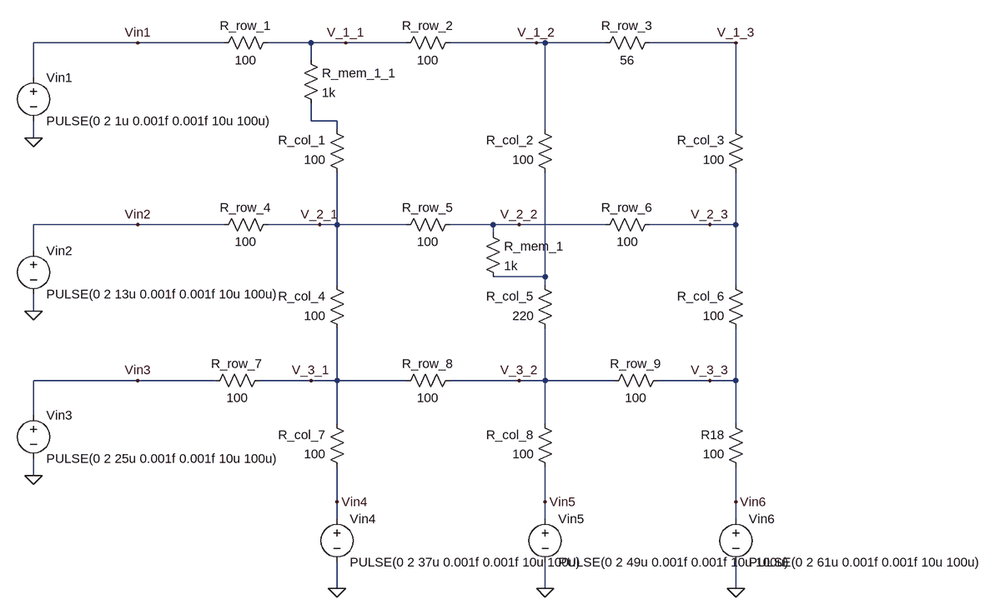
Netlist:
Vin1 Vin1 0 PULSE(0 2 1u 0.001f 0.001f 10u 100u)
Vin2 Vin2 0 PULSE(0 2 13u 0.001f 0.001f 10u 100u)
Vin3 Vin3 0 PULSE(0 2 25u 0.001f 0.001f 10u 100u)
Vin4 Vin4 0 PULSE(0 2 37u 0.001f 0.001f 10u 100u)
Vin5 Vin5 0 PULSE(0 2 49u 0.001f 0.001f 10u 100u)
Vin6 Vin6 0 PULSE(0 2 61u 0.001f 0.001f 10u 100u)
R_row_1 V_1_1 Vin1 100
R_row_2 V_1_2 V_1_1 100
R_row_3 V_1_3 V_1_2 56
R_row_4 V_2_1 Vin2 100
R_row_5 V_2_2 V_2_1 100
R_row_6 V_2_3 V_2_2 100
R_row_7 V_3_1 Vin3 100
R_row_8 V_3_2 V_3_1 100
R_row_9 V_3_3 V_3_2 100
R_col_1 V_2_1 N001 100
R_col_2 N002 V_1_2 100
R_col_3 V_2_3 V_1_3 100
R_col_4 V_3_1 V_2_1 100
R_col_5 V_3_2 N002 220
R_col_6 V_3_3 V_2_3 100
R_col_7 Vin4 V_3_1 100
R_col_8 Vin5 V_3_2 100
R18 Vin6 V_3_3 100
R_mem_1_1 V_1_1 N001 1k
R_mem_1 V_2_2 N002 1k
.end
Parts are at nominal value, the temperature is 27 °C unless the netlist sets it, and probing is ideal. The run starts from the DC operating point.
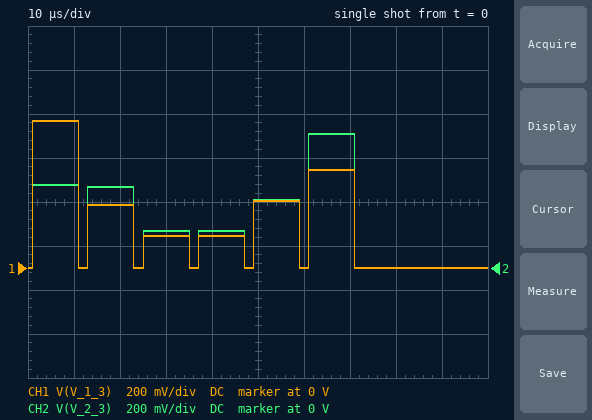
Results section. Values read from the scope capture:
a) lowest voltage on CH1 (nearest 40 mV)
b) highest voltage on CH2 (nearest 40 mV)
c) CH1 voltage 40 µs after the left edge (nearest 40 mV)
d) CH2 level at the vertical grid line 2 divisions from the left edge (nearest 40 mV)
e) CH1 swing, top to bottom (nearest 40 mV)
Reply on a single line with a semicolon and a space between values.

0 V; 600 mV; 160 mV; 360 mV; 680 mV
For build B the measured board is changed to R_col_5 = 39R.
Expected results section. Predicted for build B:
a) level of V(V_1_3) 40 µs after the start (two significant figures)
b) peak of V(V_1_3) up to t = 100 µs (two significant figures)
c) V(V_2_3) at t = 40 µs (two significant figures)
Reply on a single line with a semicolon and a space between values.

160 mV; 570 mV; 180 mV
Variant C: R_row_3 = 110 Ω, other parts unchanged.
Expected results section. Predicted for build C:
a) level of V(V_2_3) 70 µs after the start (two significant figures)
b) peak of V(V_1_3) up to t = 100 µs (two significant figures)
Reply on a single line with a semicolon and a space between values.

630 mV; 600 mV
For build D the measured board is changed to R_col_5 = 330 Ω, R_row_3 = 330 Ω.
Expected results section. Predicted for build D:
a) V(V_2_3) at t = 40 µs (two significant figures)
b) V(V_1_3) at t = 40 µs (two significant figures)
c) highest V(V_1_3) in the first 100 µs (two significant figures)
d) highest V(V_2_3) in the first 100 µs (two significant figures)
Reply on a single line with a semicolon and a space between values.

180 mV; 160 mV; 580 mV; 670 mV
